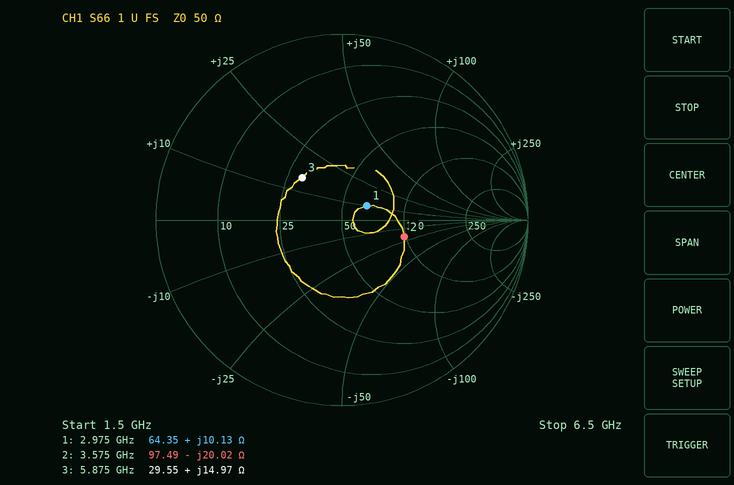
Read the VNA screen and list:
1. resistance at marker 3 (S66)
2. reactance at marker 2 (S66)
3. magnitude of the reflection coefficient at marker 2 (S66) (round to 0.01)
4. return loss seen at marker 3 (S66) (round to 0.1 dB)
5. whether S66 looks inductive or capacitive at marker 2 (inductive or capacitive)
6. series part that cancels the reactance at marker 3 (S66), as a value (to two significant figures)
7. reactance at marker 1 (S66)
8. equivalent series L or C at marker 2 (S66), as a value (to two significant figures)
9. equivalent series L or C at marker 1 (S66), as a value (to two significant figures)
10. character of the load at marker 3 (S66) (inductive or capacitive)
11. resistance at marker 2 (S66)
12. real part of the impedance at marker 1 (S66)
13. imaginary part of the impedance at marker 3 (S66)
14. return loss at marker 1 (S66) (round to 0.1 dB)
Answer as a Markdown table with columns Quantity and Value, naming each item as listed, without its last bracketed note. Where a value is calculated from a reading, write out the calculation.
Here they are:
| Quantity | Value |
|---|---|
| resistance at marker 3 | 29.55 Ω |
| reactance at marker 2 | -20.02 Ω |
| magnitude of the reflection coefficient at marker 2 (S66) | 0.35 |
| return loss seen at marker 3 (S66) | 10.1 dB |
| whether S66 looks inductive or capacitive at marker 2 | capacitive |
| series part that cancels the reactance at marker 3 (S66), as a value | C = 1/(2π × 5.875 GHz × 14.97 Ω) ≈ 1.8 pF |
| reactance at marker 1 | +10.13 Ω |
| equivalent series L or C at marker 2 (S66), as a value | C = 1/(2π × 3.575 GHz × 20.02 Ω) ≈ 2.2 pF |
| equivalent series L or C at marker 1 (S66), as a value | L = 10.13 Ω/(2π × 2.975 GHz) ≈ 542 pH, so 540 pH to two significant figures |
| character of the load at marker 3 (S66) | inductive |
| resistance at marker 2 | 97.49 Ω |
| real part of the impedance at marker 1 | 64.35 Ω |
| imaginary part of the impedance at marker 3 | +14.97 Ω |
| return loss at marker 1 (S66) | 16.3 dB |
